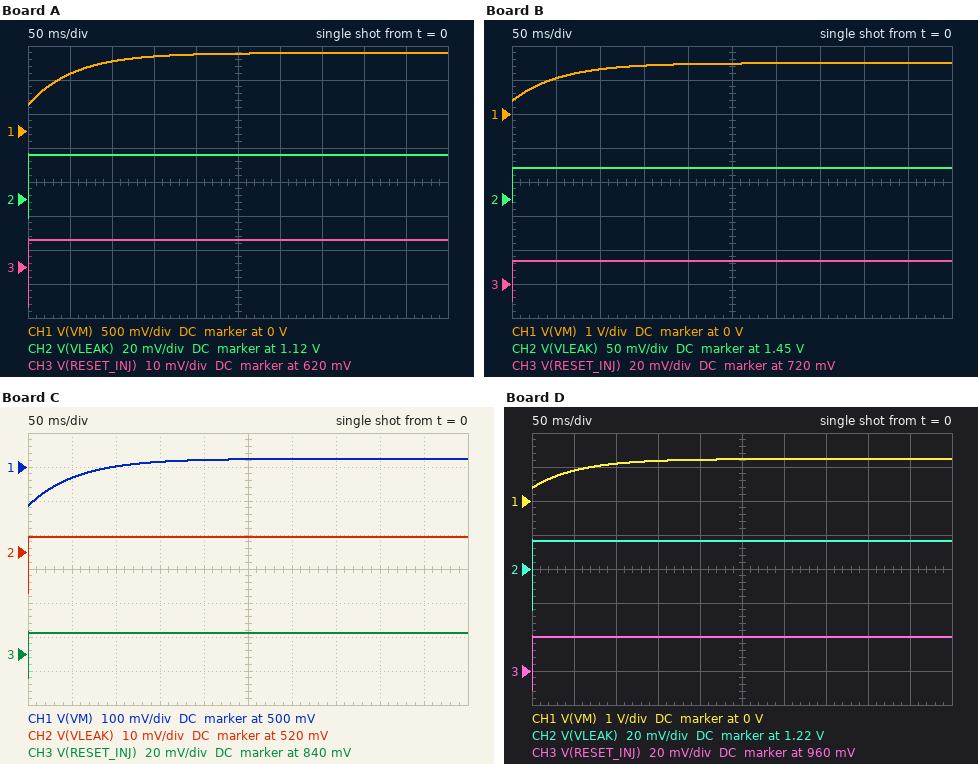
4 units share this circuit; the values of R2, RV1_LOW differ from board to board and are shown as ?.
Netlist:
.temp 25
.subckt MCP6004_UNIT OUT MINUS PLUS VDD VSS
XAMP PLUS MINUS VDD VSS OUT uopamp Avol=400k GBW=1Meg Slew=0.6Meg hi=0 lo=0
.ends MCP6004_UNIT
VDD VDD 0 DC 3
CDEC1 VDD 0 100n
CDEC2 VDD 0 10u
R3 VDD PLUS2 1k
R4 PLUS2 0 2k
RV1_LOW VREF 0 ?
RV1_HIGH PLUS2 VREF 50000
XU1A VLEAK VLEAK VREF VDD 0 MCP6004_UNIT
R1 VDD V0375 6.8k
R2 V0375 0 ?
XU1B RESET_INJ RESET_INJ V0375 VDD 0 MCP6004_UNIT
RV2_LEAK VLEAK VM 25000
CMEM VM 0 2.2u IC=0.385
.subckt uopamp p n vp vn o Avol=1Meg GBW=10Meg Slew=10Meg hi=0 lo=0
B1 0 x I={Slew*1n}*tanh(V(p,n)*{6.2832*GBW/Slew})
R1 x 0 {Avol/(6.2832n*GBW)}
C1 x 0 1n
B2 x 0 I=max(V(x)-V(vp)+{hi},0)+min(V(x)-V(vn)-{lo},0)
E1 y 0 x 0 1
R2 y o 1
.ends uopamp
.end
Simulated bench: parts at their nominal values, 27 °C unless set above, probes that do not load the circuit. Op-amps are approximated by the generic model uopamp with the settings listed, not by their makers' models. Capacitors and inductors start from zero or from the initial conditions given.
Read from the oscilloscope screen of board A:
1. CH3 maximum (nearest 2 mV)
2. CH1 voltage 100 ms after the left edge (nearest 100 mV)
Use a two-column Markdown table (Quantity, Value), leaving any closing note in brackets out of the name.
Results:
| Quantity | Value |
|---|---|
| CH3 maximum | 628 mV |
| CH1 voltage 100 ms after the left edge | 1.0 V |
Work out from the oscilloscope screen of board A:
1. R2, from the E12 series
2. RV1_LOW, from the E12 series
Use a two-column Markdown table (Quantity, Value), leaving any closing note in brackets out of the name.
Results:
| Quantity | Value |
|---|---|
| R2, from the E12 series | 1.8 kΩ |
| RV1_LOW, from the E12 series | 68 kΩ |
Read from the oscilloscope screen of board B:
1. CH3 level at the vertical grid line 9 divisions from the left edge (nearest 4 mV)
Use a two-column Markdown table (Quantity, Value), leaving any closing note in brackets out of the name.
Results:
| Quantity | Value |
|---|---|
| CH3 level at the vertical grid line 9 divisions from the left edge | 732 mV |
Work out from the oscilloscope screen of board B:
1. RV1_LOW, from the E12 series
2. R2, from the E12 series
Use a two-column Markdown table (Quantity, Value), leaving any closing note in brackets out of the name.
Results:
| Quantity | Value |
|---|---|
| RV1_LOW, from the E12 series | 150 kΩ |
| R2, from the E12 series | 2.2 kΩ |
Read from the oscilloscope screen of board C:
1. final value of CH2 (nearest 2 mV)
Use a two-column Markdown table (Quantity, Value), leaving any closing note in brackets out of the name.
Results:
| Quantity | Value |
|---|---|
| final value of CH2 | 524 mV |
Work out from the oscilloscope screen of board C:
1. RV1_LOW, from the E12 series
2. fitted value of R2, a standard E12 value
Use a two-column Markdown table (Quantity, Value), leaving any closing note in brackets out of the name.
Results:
| Quantity | Value |
|---|---|
| RV1_LOW, from the E12 series | 18 kΩ |
| fitted value of R2, a standard E12 value | 2.7 kΩ |
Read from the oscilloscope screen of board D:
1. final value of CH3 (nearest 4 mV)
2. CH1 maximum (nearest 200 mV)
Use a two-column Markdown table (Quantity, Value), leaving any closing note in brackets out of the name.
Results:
| Quantity | Value |
|---|---|
| final value of CH3 | 980 mV |
| CH1 maximum | 1.2 V |
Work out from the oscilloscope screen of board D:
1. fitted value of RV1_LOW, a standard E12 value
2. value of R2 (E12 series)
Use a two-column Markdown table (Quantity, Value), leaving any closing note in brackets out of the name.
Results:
| Quantity | Value |
|---|---|
| fitted value of RV1_LOW, a standard E12 value | 82 kΩ |
| value of R2 | 3.3 kΩ |
